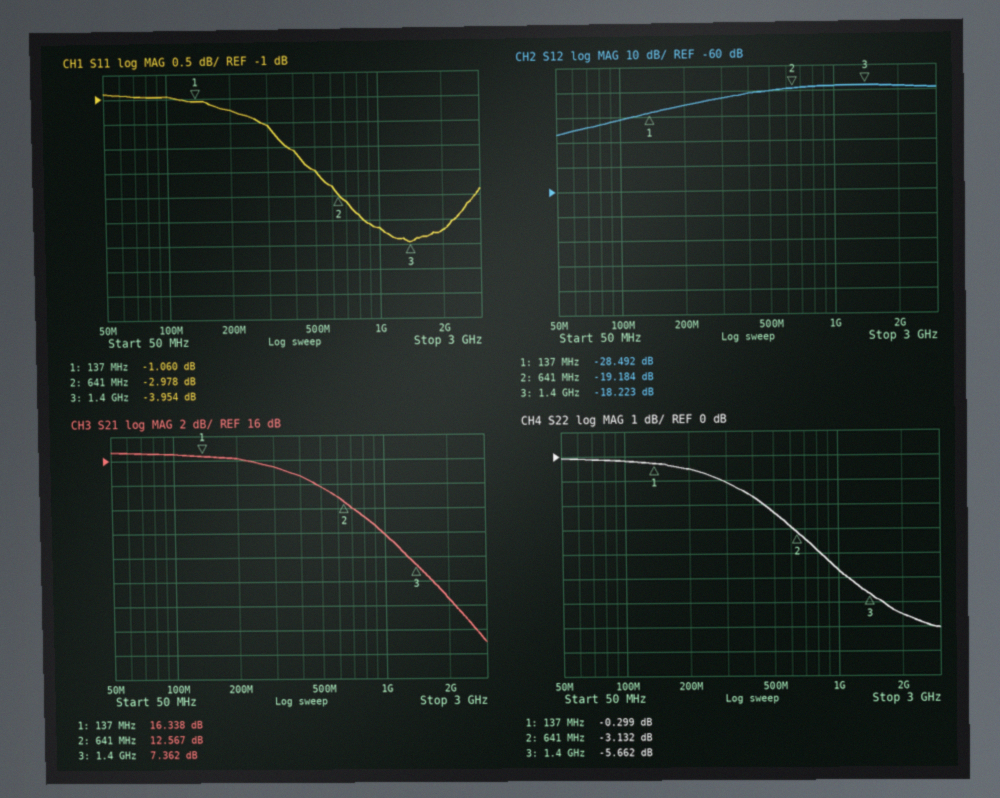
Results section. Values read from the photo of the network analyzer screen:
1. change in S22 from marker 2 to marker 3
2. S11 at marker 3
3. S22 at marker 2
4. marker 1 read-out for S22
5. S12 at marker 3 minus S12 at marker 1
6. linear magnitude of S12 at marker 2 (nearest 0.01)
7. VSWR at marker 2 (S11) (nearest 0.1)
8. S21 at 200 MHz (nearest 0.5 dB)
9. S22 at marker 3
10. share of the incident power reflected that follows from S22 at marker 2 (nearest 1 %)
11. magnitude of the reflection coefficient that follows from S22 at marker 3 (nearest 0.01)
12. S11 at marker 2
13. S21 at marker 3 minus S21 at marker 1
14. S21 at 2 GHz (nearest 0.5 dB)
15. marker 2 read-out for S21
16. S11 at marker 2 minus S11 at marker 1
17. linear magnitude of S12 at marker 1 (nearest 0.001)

-2.530 dB
-3.954 dB
-3.132 dB
-0.299 dB
10.269 dB
0.11
5.9
16.0 dB
-5.662 dB
49 %
0.52
-2.978 dB
-8.976 dB
4.5 dB
12.567 dB
-1.918 dB
0.038
